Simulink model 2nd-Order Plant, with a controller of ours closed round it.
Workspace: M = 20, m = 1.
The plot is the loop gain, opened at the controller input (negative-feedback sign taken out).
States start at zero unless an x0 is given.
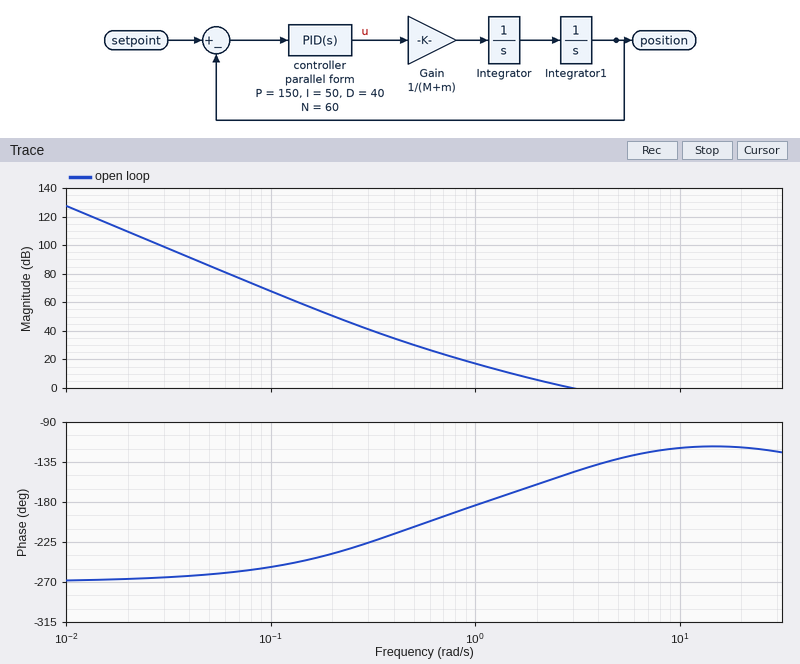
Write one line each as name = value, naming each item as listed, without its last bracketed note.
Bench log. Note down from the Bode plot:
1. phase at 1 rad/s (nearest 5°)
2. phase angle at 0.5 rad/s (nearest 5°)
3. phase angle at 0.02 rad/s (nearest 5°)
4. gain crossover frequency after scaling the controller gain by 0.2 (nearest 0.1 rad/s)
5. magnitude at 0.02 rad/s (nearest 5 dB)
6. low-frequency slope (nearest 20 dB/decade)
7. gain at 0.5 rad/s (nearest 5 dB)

phase at 1 rad/s = -185°
phase angle at 0.5 rad/s = -210°
phase angle at 0.02 rad/s = -265°
gain crossover frequency after scaling the controller gain by 0.2 = 1.2 rad/s
magnitude at 0.02 rad/s = 110 dB
low-frequency slope = -60 dB/decade
gain at 0.5 rad/s = 30 dB
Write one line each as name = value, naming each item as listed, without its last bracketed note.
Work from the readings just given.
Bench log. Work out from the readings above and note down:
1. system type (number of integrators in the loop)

system type = 3
